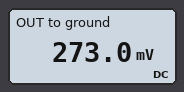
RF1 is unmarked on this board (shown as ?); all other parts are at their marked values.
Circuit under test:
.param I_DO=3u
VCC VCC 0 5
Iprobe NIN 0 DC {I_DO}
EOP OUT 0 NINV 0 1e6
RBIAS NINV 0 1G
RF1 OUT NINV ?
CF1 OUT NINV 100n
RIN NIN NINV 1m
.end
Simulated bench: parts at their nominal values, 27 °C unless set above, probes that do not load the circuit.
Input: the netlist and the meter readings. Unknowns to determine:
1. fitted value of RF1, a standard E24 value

91 kΩ
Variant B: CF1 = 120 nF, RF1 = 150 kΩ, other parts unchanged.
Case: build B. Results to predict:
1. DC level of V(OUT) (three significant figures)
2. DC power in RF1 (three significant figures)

450 mV
1.35 µW
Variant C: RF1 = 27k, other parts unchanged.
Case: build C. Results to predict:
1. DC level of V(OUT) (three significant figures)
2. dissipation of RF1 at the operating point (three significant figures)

81.0 mV
243 nW
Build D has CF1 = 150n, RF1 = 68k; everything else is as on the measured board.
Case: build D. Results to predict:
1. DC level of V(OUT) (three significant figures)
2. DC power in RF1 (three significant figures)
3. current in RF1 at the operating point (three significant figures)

204 mV
612 nW
3.00 µA
